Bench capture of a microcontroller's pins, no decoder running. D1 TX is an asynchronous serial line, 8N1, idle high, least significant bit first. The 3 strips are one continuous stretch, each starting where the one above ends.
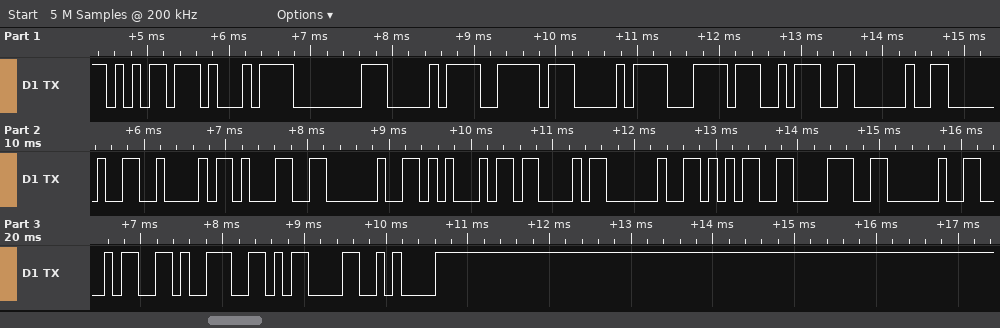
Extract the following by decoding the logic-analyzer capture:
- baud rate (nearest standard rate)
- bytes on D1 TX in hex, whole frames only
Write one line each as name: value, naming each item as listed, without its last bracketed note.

baud rate: 9600 baud
bytes on D1 TX in hex, whole frames only: B5 D1 80 D0 BE D0 BC 3A 20 20 42 31 20 45 43 20 35 38 20 34 39 0D 0A
